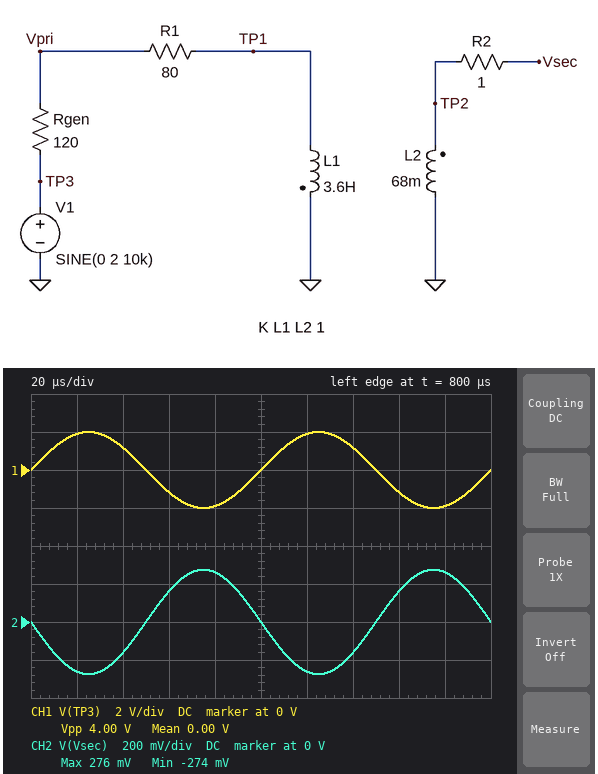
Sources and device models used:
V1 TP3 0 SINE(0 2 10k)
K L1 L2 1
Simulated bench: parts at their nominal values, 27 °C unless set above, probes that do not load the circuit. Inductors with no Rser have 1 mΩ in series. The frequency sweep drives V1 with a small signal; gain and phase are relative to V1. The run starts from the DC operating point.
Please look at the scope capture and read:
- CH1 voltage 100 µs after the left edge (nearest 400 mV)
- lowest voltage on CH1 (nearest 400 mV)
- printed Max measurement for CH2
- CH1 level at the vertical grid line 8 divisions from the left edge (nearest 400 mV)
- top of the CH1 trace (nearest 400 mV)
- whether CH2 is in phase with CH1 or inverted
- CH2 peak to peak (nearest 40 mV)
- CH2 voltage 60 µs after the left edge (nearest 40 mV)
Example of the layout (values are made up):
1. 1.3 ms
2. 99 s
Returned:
1. 0 V
2. -2.0 V
3. 276 mV
4. -1.2 V
5. 2.0 V
6. inverted
7. 560 mV
8. 160 mV
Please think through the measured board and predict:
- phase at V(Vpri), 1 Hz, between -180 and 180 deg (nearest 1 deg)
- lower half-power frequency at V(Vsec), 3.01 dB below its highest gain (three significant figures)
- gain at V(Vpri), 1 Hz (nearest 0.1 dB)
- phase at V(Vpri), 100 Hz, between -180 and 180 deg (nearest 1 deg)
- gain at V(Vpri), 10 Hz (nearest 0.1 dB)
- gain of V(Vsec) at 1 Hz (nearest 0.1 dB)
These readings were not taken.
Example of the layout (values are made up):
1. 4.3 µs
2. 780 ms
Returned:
1. 9 deg
2. 8.84 Hz
3. -7.7 dB
4. 3 deg
5. -2.0 dB
6. -36.2 dB
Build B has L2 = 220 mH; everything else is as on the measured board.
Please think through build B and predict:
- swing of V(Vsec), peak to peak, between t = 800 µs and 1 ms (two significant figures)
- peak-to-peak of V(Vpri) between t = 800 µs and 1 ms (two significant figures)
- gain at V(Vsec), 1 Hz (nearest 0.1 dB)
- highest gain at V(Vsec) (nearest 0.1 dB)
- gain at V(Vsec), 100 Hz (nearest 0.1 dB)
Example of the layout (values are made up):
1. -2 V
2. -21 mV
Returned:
1. 990 mV
2. 4.0 V
3. -31.1 dB
4. -12.1 dB
5. -12.2 dB
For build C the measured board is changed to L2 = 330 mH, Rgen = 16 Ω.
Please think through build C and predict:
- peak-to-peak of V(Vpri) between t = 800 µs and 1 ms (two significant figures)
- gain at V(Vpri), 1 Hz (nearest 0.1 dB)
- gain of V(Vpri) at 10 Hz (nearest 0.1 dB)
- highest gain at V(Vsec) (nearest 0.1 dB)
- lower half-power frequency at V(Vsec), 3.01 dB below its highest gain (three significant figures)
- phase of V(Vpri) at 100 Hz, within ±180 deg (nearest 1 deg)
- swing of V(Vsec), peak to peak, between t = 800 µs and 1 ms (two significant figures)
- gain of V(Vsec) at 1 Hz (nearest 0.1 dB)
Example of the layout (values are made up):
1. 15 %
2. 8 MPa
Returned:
1. 4.0 V
2. -1.5 dB
3. -0.2 dB
4. -10.4 dB
5. 4.24 Hz
6. 0 deg
7. 1.2 V
8. -23.2 dB
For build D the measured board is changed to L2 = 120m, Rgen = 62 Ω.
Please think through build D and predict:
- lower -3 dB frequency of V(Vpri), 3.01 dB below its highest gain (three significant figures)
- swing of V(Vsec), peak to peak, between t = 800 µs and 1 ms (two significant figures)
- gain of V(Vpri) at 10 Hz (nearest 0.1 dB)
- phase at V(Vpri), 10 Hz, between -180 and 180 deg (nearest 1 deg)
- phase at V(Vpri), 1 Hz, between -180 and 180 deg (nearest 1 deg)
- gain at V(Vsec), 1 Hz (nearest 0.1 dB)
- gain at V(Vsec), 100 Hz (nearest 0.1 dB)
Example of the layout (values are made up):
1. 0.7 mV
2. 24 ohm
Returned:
1. 3.79 Hz
2. 730 mV
3. -0.9 dB
4. 13 deg
5. 7 deg
6. -30.8 dB
7. -14.8 dB
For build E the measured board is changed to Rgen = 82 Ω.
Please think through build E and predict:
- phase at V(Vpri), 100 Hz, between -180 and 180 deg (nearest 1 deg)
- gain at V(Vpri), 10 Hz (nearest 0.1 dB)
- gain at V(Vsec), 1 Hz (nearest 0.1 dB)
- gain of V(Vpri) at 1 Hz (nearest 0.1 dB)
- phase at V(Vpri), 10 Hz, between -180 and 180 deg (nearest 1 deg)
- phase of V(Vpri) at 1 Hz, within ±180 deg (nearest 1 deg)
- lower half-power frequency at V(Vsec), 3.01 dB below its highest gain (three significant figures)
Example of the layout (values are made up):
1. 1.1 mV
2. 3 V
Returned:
1. 2 deg
2. -1.3 dB
3. -34.4 dB
4. -5.9 dB
5. 16 deg
6. 8 deg
7. 7.16 Hz
